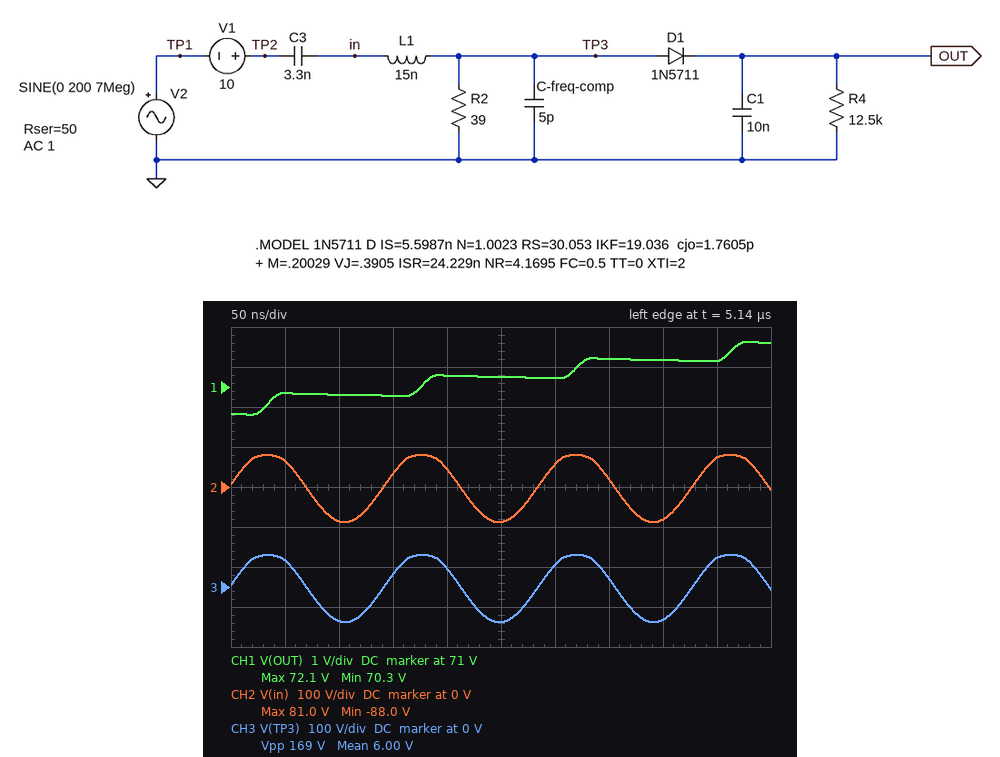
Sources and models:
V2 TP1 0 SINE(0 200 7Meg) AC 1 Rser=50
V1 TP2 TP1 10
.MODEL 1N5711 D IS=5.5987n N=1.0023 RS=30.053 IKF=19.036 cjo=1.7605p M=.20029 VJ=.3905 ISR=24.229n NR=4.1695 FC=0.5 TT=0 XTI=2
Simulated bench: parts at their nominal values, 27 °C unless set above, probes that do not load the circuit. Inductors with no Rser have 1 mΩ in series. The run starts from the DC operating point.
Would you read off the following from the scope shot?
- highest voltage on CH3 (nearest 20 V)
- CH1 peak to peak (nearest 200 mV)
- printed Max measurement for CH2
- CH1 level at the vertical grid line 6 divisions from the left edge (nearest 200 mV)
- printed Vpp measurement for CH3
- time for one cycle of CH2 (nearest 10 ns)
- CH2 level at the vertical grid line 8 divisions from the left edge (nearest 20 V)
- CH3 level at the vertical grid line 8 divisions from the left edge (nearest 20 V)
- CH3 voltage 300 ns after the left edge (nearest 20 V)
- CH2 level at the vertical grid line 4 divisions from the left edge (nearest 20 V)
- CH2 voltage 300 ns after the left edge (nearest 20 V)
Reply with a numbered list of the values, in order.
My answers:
1. 80 V
2. 1.8 V
3. 81.0 V
4. 71.2 V
5. 169 V
6. 140 ns
7. -80 V
8. -80 V
9. 60 V
10. 40 V
11. 60 V
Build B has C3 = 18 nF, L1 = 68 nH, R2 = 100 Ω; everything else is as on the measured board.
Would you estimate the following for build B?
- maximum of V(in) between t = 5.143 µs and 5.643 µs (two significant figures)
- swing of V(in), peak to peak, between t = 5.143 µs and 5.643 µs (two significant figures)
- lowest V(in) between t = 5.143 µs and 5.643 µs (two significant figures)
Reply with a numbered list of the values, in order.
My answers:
1. 110 V
2. 250 V
3. -140 V
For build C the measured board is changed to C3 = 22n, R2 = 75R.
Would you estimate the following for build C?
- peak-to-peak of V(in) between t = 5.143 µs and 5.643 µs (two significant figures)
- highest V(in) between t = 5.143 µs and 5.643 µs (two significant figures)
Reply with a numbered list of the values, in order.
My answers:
1. 230 V
2. 100 V
